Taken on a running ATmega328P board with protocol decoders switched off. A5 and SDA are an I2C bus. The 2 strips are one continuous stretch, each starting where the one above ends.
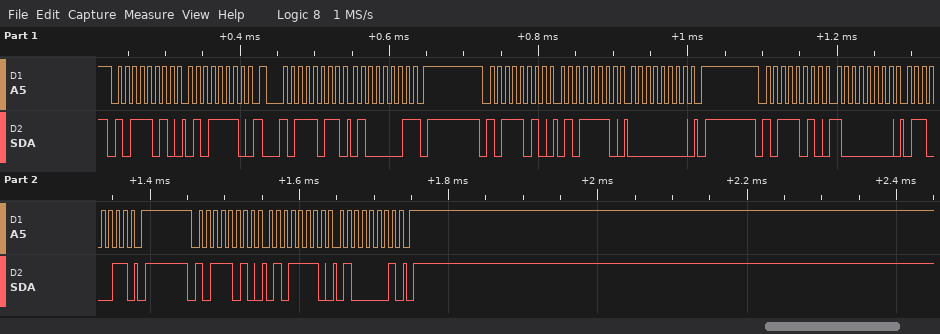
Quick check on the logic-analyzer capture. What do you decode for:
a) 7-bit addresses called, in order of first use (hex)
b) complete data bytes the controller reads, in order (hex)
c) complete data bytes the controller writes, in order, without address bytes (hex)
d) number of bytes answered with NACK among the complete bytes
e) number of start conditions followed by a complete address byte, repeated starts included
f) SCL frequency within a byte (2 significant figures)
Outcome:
0x5D
41
5E 5E 00 80 63 5E 41
1
5
100 kHz
